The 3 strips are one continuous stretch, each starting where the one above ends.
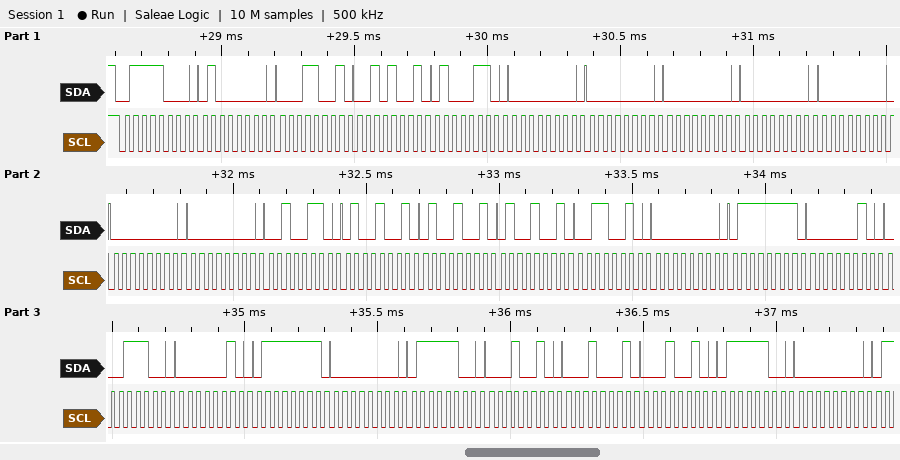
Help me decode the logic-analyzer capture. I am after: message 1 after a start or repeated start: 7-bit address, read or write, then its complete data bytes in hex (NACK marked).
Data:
0x3C write: 40 19 29 46 00 00 00 00 00 00 00 26 49 49 49 32 00 7F 02 1C 02 7F 00 7C 12 11 12 7C 00
